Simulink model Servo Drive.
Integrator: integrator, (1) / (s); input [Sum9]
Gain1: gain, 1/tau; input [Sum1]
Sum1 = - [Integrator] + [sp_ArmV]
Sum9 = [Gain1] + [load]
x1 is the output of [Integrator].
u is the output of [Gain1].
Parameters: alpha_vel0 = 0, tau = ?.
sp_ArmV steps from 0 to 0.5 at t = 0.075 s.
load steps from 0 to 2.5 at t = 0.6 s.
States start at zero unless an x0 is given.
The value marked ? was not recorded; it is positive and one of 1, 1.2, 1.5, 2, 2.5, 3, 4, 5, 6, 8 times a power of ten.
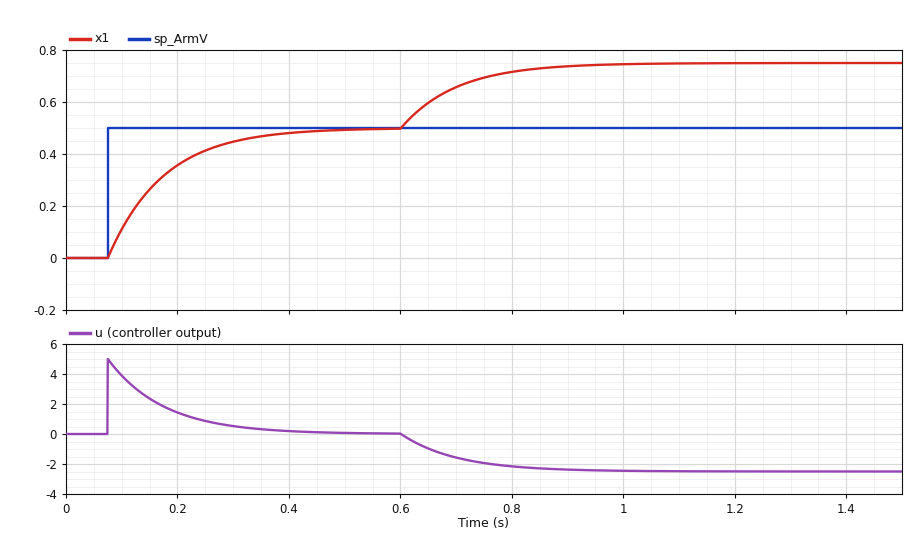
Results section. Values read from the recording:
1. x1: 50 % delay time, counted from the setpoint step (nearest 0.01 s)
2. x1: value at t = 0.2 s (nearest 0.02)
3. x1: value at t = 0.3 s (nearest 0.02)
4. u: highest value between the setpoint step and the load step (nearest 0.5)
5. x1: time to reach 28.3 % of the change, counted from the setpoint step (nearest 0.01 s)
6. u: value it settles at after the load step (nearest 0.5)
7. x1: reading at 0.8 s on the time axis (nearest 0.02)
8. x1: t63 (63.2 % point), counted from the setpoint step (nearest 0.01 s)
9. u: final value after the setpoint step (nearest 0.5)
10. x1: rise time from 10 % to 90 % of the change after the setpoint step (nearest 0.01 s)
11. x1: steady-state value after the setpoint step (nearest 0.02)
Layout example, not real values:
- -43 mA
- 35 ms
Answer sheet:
- 0.07 s
- 0.36
- 0.44
- 5.0
- 0.03 s
- -2.5
- 0.72
- 0.10 s
- 0.0
- 0.22 s
- 0.50
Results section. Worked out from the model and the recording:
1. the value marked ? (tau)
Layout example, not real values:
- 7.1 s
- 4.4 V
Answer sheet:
- 0.1
